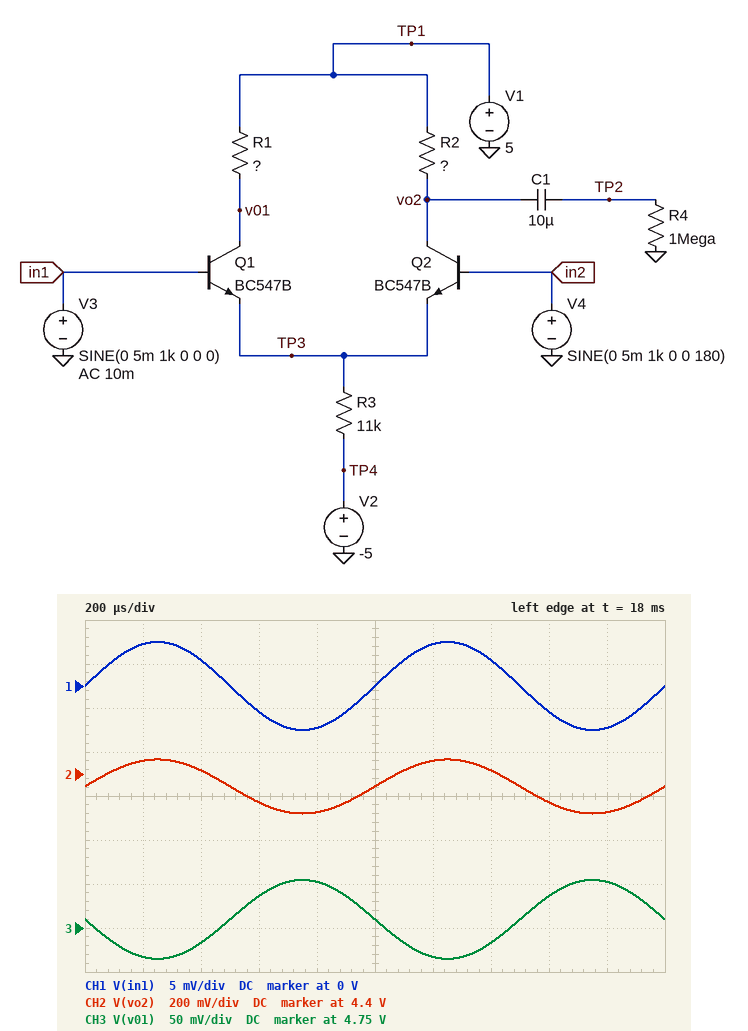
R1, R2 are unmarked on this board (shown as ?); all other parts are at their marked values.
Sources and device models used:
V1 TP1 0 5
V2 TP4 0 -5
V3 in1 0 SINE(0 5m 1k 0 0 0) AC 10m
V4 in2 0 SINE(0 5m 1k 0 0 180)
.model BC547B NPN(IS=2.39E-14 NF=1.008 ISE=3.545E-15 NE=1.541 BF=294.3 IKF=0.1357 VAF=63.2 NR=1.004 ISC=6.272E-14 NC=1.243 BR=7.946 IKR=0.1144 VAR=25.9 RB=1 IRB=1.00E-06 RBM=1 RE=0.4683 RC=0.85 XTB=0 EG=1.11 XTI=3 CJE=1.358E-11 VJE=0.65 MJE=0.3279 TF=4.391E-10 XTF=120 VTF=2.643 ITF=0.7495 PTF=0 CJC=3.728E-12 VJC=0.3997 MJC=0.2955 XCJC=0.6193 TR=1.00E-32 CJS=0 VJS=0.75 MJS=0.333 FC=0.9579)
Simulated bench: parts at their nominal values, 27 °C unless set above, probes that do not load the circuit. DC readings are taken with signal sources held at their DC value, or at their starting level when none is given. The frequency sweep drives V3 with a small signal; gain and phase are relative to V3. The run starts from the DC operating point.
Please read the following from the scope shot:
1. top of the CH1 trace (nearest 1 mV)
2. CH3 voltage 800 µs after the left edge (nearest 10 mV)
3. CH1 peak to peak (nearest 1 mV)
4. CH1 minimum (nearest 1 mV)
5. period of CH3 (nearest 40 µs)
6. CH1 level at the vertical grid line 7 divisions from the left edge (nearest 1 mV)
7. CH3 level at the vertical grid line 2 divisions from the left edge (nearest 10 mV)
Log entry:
5 mV
4.80 V
10 mV
-5 mV
1.00 ms
3 mV
4.73 V
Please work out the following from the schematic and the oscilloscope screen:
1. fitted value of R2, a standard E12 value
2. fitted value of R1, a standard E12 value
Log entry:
3.3 kΩ
1.2 kΩ
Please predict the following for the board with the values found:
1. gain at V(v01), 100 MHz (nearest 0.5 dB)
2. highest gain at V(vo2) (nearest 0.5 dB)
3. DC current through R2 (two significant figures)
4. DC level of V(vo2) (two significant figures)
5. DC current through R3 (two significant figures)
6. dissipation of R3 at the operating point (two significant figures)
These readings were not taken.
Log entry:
9.0 dB
22.0 dB
200 µA
4.3 V
400 µA
1.8 mW
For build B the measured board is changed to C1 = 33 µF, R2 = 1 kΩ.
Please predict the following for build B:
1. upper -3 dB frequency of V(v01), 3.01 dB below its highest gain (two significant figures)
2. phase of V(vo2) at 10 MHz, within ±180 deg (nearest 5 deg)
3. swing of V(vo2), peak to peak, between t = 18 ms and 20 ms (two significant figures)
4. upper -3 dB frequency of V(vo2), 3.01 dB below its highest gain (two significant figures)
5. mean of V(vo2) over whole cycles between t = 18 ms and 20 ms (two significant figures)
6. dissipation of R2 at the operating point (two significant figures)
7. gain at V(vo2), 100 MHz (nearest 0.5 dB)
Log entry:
79 MHz
-5 deg
75 mV
92 MHz
4.8 V
40 µW
8.0 dB
